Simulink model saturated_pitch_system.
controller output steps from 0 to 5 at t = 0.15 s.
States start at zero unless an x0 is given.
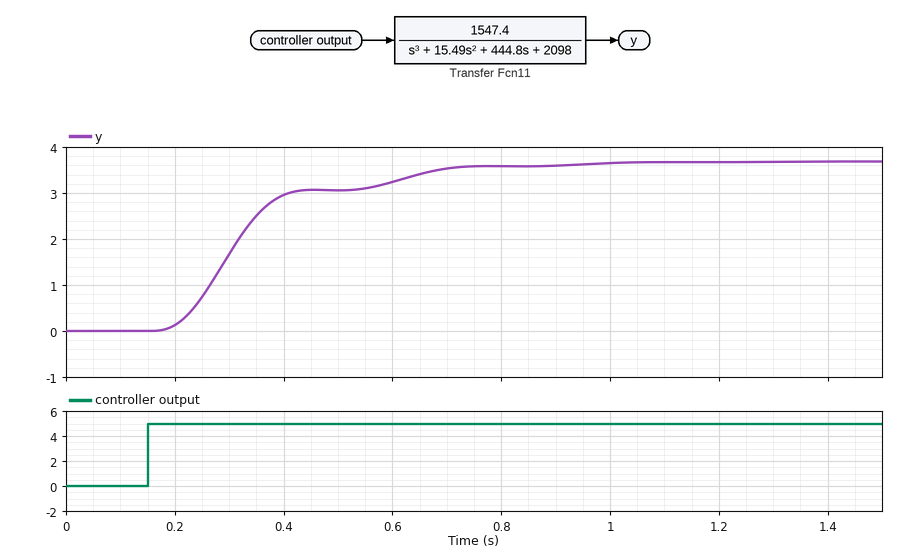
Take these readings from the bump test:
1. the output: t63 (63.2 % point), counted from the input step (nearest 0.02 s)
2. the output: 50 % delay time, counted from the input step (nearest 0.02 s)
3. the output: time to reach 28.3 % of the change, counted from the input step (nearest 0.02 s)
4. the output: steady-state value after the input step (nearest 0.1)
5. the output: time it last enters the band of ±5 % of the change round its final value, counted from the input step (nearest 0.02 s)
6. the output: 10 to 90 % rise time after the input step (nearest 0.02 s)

0.18 s
0.16 s
0.12 s
3.7
0.54 s
0.40 s
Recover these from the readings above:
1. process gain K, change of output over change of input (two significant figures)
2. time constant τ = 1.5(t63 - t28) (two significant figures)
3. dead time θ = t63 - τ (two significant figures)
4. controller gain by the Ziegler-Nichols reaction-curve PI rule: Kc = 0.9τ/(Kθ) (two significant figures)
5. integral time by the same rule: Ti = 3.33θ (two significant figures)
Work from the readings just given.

0.74
0.090 s
0.090 s
1.2
0.30 s
